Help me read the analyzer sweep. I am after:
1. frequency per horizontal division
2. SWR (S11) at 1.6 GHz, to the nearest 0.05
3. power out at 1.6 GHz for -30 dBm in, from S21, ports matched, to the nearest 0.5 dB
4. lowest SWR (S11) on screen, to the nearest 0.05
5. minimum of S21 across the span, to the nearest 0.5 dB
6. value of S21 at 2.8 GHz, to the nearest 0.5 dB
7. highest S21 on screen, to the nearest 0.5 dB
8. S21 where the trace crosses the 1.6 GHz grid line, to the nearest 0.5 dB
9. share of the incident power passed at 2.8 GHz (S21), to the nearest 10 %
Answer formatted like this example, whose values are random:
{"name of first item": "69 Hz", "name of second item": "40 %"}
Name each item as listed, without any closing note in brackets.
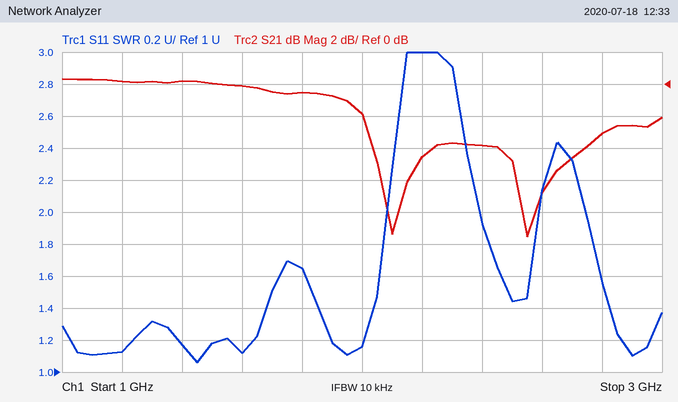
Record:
{"frequency per horizontal division": "200 MHz", "SWR (S11) at 1.6 GHz, to the nearest 0.05": "1.10", "power out at 1.6 GHz for -30 dBm in, from S21, ports matched, to the nearest 0.5 dB": "-30.0 dBm", "lowest SWR (S11) on screen, to the nearest 0.05": "1.05", "minimum of S21 across the span, to the nearest 0.5 dB": "-9.5 dB", "value of S21 at 2.8 GHz, to the nearest 0.5 dB": "-3.0 dB", "highest S21 on screen, to the nearest 0.5 dB": "0.5 dB", "S21 where the trace crosses the 1.6 GHz grid line, to the nearest 0.5 dB": "0.0 dB", "share of the incident power passed at 2.8 GHz (S21), to the nearest 10 %": "50 %"}
